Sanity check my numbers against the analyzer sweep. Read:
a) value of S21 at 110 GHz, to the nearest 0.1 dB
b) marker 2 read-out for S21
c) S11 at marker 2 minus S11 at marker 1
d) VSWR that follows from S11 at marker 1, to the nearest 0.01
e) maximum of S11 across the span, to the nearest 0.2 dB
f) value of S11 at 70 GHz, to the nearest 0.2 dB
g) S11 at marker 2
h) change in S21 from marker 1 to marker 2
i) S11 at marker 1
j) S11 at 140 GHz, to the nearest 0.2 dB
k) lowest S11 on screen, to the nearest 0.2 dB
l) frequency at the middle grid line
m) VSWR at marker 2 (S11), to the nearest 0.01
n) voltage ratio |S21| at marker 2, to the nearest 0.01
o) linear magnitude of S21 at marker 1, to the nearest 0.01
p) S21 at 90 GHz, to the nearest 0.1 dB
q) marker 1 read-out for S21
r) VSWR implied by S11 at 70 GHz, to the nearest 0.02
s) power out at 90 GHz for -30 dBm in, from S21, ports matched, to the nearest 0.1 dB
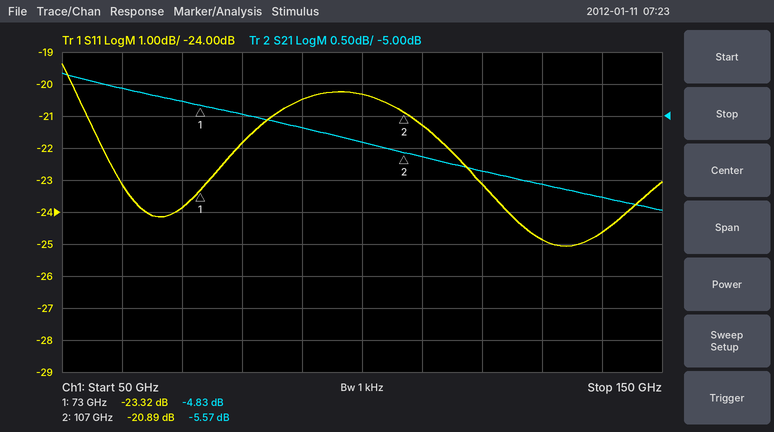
-5.6 dB
-5.57 dB
2.43 dB
1.15
-19.4 dB
-23.8 dB
-20.89 dB
-0.74 dB
-23.32 dB
-24.6 dB
-25.0 dB
100 GHz
1.20
0.53
0.57
-5.2 dB
-4.83 dB
1.14
-35.2 dBm
